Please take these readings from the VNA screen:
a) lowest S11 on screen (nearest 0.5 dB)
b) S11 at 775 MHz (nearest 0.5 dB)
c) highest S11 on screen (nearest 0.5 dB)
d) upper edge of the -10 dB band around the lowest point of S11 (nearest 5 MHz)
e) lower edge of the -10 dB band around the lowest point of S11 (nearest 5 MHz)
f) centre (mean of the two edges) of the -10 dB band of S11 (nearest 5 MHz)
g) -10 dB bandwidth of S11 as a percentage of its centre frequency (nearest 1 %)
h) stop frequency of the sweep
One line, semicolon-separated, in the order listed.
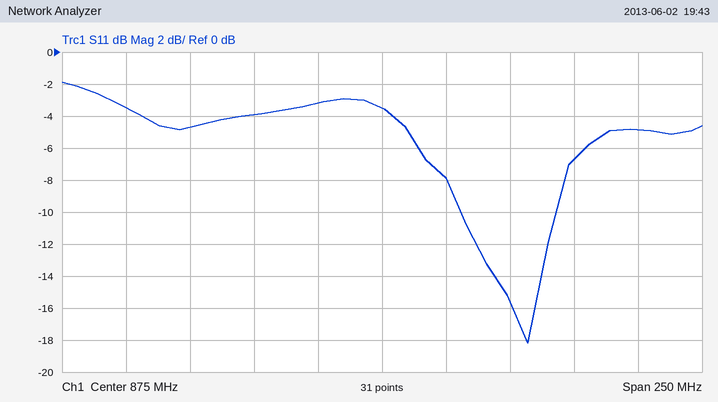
-18.0 dB; -3.5 dB; -2.0 dB; 945 MHz; 905 MHz; 925 MHz; 4 %; 1 GHz
